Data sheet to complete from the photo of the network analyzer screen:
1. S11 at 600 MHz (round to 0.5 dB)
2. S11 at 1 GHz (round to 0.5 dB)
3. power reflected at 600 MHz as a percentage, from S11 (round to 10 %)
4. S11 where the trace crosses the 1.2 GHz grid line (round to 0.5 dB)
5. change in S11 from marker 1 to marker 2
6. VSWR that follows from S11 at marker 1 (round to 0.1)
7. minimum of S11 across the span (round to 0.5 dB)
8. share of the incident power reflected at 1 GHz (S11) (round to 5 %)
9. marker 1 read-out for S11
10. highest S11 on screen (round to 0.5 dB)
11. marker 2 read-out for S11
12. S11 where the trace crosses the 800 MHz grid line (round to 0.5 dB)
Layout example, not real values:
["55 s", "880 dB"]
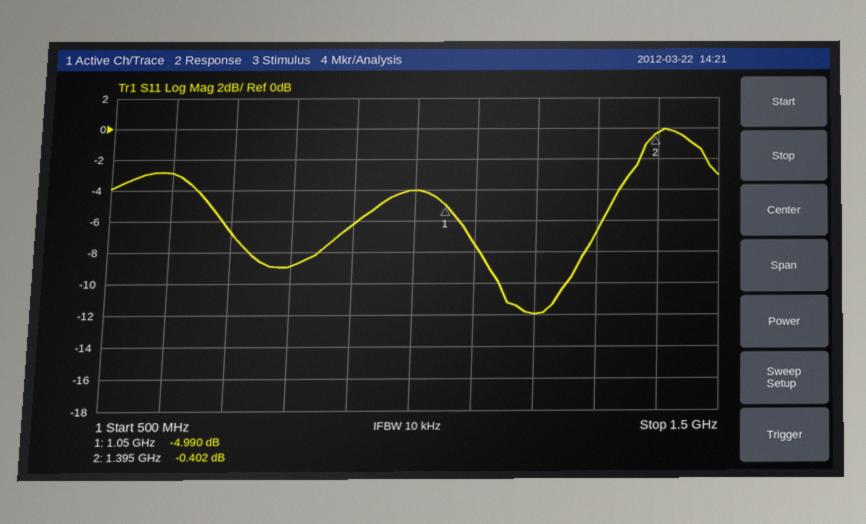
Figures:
["-3.0 dB", "-4.0 dB", "50 %", "-12.0 dB", "4.588 dB", "3.6", "-12.0 dB", "40 %", "-4.990 dB", "0.0 dB", "-0.402 dB", "-9.0 dB"]
